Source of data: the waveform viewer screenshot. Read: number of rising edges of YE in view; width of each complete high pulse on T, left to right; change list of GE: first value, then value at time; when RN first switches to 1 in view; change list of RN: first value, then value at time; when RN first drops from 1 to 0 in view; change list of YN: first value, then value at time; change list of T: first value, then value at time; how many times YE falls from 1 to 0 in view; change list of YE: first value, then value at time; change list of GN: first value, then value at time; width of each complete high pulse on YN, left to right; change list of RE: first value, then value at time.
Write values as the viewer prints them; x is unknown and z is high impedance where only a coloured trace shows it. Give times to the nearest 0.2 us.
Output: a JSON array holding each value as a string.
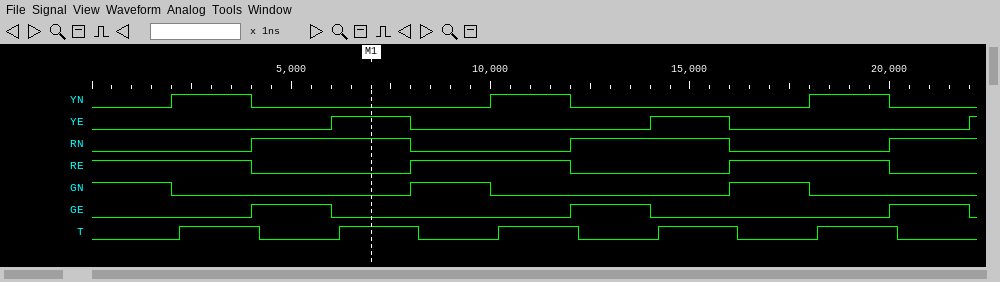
["3", "2 us, 2 us, 2 us, 2 us, 2 us", "0, 1 at 4 us, 0 at 6 us, 1 at 12 us, 0 at 14 us, 1 at 20 us, 0 at 22 us", "4 us", "0, 1 at 4 us, 0 at 8 us, 1 at 12 us, 0 at 16 us, 1 at 20 us", "8 us", "0, 1 at 2 us, 0 at 4 us, 1 at 10 us, 0 at 12 us, 1 at 18 us, 0 at 20 us", "0, 1 at 2.2 us, 0 at 4.2 us, 1 at 6.2 us, 0 at 8.2 us, 1 at 10.2 us, 0 at 12.2 us, 1 at 14.2 us, 0 at 16.2 us, 1 at 18.2 us, 0 at 20.2 us", "2", "0, 1 at 6 us, 0 at 8 us, 1 at 14 us, 0 at 16 us, 1 at 22 us", "1, 0 at 2 us, 1 at 8 us, 0 at 10 us, 1 at 16 us, 0 at 18 us", "2 us, 2 us, 2 us", "1, 0 at 4 us, 1 at 8 us, 0 at 12 us, 1 at 16 us, 0 at 20 us"]
